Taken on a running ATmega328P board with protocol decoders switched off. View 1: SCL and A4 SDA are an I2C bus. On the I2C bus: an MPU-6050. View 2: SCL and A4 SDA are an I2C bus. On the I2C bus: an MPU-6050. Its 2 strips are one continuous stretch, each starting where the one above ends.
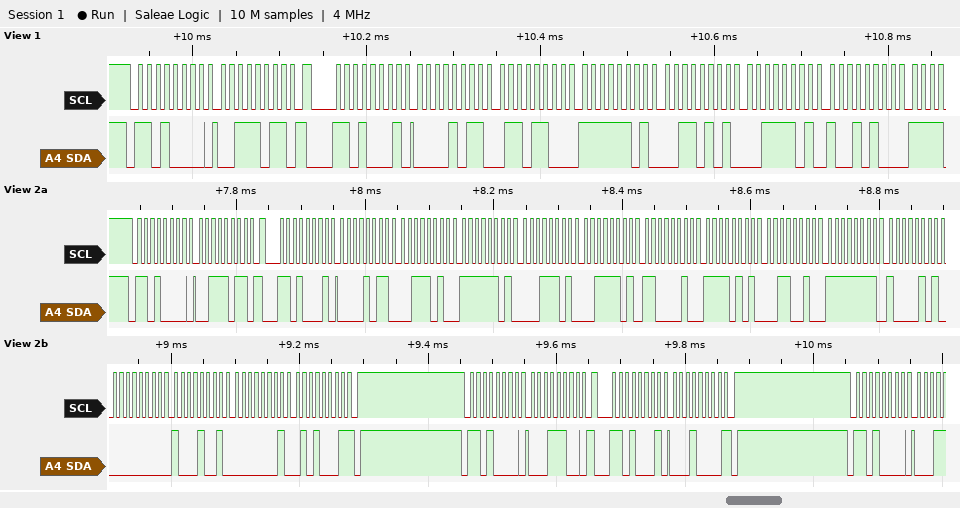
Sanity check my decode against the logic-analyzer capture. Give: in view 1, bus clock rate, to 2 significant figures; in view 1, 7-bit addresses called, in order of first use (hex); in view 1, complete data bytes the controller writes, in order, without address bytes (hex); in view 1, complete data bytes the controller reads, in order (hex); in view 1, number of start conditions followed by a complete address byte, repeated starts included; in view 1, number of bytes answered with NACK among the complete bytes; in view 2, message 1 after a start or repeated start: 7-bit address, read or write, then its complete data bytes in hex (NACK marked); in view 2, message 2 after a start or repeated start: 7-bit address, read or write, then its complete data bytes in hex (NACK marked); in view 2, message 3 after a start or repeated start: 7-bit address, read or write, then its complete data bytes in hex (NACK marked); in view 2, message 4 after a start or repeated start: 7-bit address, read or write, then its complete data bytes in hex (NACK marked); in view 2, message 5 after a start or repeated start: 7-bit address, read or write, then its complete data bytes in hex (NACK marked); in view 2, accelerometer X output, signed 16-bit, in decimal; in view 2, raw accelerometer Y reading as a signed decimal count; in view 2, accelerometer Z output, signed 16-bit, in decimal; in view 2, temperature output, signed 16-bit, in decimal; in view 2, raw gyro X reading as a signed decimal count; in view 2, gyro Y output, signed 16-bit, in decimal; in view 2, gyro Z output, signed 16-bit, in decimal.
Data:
100 kHz
0x68
3B
0B 6C FD 35 3D 94
2
0
0x68 write: 3B
0x68 read: 0B 3A FD 1D 3D C2 F5 32 FF 85 00 89 01 51 NACK
0x68 write: 1C
0x68 read: 10 NACK
0x68 write
2874
-739
15810
-2766
-123
137
337
